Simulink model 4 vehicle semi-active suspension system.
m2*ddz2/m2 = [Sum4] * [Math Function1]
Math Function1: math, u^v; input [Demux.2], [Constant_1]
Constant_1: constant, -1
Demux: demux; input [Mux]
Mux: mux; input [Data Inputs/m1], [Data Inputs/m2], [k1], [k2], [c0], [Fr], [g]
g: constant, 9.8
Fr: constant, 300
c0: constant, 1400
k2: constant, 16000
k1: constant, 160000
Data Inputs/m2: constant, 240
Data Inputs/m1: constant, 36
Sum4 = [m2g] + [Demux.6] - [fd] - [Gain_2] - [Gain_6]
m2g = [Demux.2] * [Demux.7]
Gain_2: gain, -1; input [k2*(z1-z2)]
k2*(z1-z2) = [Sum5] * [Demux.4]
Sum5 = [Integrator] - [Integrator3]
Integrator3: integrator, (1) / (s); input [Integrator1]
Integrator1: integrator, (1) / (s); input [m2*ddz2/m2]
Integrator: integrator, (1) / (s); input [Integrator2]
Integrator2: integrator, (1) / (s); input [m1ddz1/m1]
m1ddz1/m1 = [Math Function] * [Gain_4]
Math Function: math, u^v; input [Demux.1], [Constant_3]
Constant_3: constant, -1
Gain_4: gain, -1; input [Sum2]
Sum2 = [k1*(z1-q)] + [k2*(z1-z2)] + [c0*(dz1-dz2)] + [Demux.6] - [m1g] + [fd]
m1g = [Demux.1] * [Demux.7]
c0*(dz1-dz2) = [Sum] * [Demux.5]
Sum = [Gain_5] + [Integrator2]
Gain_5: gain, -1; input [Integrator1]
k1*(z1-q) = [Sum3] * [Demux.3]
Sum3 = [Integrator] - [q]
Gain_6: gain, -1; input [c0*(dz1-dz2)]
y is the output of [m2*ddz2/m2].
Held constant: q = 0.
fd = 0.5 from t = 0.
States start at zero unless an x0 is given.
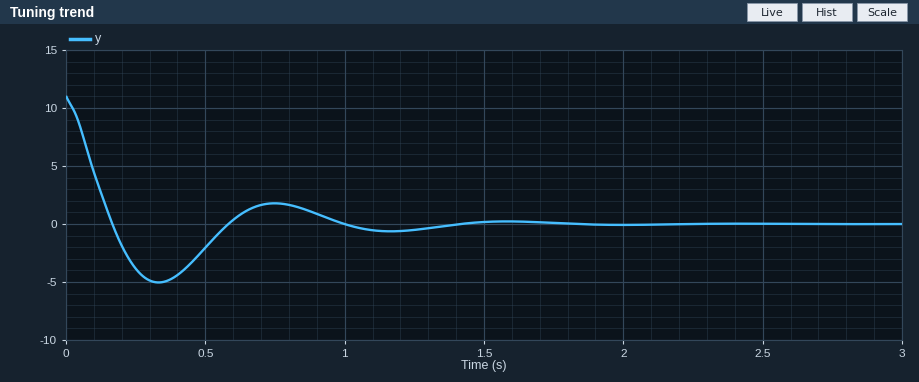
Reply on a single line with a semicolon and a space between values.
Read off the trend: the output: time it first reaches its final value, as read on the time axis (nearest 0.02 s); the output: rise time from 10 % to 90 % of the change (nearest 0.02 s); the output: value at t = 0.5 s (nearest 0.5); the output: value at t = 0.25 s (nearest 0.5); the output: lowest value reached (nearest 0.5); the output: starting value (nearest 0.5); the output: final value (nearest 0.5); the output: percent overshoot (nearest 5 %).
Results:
0.16 s; 0.12 s; -2.0; -4.0; -5.0; 11.0; 0.0; 45 %
